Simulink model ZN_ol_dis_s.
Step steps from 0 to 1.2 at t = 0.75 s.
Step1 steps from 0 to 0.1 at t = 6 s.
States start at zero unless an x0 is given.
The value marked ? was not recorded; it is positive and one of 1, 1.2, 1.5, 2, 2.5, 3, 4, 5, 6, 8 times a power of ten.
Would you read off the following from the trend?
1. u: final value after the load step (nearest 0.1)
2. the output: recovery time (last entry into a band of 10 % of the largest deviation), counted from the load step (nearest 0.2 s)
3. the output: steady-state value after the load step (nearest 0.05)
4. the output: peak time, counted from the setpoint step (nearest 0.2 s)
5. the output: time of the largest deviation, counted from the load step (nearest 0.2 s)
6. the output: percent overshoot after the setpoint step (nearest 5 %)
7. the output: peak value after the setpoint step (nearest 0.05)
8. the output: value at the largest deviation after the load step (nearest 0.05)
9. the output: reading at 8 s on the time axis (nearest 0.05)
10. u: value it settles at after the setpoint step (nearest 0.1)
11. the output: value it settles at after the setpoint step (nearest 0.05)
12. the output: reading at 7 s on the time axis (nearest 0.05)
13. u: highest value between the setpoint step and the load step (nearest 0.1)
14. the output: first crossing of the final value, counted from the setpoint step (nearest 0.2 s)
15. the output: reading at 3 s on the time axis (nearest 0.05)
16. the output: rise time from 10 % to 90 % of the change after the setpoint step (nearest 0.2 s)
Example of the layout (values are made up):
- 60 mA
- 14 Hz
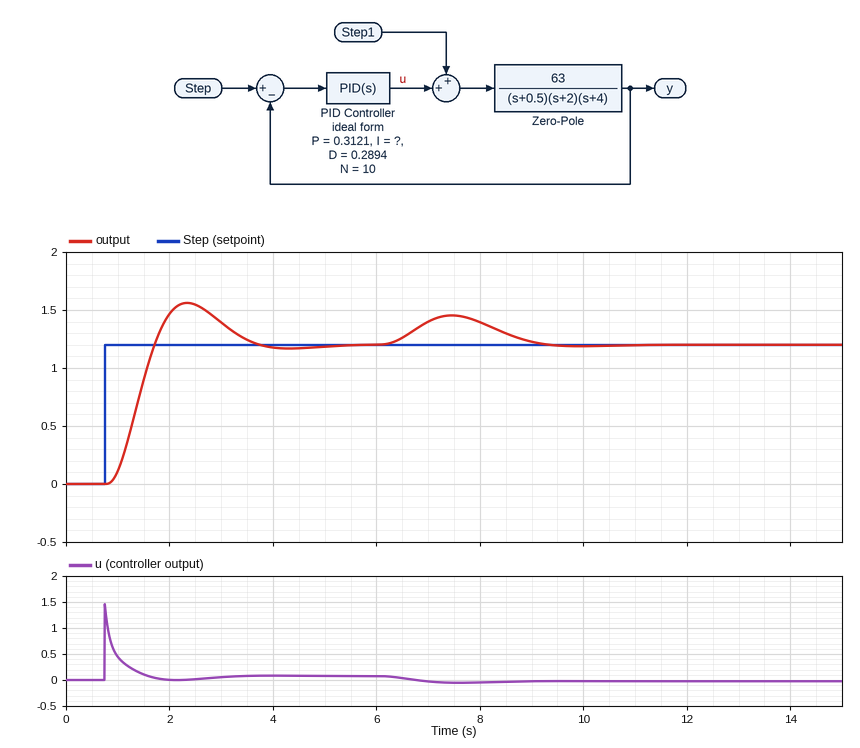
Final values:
- 0.0
- 3.0 s
- 1.20
- 1.6 s
- 1.4 s
- 30 %
- 1.55
- 1.45
- 1.40
- 0.1
- 1.20
- 1.40
- 1.5
- 1.0 s
- 1.40
- 0.6 s
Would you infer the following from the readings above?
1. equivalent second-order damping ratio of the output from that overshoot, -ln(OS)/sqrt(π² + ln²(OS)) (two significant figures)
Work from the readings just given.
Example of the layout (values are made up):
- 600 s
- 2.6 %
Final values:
- 0.36
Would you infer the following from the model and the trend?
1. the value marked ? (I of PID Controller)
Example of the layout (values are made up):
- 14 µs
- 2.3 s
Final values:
- 0.8
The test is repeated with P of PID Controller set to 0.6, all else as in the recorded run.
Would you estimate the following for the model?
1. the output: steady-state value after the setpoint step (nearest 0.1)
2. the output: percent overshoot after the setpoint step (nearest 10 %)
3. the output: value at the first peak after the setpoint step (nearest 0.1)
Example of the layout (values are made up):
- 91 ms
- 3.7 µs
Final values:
- 1.2
- 50 %
- 1.8
